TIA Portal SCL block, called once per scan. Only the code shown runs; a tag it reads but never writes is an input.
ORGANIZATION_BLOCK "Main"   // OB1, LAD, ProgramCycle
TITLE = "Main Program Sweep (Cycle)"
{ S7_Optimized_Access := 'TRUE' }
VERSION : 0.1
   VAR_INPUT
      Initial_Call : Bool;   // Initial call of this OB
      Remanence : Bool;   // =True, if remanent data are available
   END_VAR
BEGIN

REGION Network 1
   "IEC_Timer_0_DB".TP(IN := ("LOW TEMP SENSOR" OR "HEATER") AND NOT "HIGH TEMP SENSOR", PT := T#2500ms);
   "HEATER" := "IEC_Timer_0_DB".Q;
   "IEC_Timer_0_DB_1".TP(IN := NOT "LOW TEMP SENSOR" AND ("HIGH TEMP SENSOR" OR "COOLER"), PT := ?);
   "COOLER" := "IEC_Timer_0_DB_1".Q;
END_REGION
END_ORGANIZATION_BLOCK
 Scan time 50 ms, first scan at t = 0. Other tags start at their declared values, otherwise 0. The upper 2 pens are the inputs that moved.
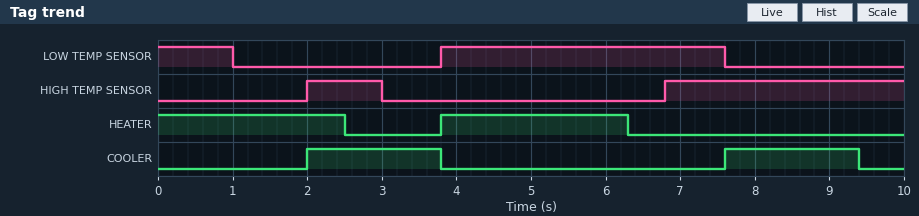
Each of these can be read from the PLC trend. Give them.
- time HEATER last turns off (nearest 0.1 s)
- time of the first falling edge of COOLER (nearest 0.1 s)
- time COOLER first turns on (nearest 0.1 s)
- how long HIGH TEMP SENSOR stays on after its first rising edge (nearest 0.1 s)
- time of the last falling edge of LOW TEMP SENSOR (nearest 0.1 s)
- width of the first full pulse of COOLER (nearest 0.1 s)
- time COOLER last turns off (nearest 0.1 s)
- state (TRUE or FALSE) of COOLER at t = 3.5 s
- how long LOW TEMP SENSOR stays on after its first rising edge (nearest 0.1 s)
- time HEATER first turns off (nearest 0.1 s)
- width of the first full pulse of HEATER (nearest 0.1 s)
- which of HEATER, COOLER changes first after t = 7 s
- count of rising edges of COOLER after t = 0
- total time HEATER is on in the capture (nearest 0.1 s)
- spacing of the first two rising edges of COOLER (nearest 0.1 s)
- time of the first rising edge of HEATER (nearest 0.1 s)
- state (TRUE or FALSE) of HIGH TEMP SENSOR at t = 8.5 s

6.3 s
3.8 s
2.0 s
1.0 s
7.6 s
1.8 s
9.4 s
TRUE
3.8 s
2.5 s
2.5 s
COOLER
2
5.0 s
5.6 s
3.8 s
TRUE
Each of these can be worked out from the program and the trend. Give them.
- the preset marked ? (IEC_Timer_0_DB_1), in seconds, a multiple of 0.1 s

1.8 s
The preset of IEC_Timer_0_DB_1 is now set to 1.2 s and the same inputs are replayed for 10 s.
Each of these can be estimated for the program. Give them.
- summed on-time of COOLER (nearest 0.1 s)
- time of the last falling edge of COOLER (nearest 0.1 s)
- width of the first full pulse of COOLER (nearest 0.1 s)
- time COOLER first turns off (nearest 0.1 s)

2.4 s
8.8 s
1.2 s
3.2 s
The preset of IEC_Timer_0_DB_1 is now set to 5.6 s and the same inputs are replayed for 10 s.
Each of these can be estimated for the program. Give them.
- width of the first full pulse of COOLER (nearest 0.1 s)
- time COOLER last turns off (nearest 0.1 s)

5.6 s
7.6 s
